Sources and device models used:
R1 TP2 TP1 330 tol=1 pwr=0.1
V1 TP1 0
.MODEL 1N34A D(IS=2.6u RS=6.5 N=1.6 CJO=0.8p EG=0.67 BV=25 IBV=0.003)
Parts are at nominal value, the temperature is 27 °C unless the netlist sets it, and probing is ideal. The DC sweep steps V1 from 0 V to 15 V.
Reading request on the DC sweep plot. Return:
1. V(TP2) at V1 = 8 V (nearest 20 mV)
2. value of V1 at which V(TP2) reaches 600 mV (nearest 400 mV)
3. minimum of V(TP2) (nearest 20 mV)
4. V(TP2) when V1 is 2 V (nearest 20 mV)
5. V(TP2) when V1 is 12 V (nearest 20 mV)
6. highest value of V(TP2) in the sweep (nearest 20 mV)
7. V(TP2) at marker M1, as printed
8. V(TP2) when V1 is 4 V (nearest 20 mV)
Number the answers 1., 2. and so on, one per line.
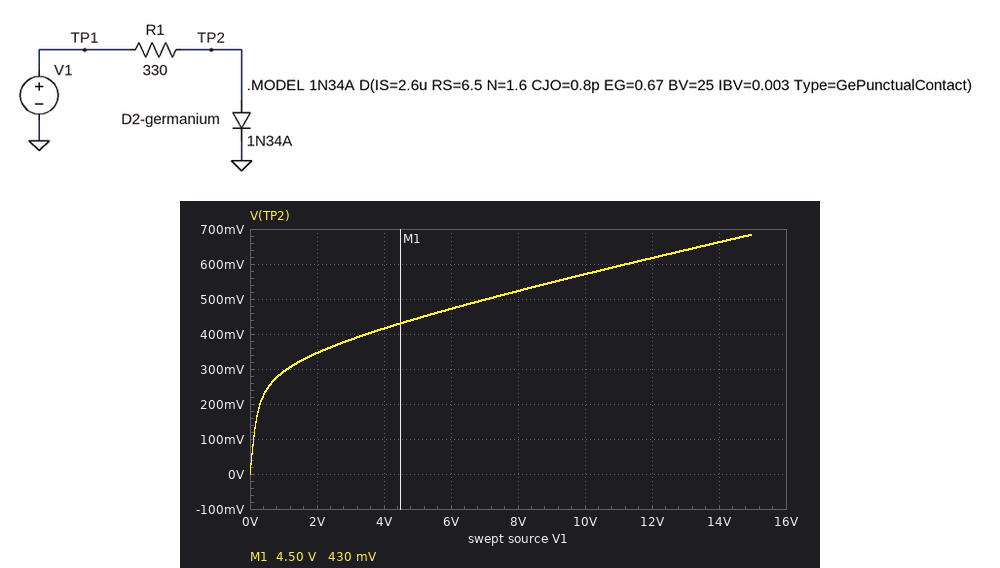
1. 520 mV
2. 11.2 V
3. 0 V
4. 340 mV
5. 620 mV
6. 680 mV
7. 430 mV
8. 420 mV
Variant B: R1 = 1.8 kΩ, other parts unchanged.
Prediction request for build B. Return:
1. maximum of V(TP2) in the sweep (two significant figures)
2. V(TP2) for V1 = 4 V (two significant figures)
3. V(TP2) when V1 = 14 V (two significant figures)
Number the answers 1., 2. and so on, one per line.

1. 390 mV
2. 290 mV
3. 380 mV
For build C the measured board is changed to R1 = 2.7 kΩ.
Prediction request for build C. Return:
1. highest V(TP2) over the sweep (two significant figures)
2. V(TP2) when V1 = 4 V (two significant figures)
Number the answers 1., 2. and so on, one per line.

1. 350 mV
2. 270 mV
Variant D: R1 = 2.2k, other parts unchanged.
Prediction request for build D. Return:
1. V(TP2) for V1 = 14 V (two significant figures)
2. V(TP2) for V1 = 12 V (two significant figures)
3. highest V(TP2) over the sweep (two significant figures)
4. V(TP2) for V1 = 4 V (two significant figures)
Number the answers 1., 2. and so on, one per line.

1. 360 mV
2. 350 mV
3. 370 mV
4. 280 mV
